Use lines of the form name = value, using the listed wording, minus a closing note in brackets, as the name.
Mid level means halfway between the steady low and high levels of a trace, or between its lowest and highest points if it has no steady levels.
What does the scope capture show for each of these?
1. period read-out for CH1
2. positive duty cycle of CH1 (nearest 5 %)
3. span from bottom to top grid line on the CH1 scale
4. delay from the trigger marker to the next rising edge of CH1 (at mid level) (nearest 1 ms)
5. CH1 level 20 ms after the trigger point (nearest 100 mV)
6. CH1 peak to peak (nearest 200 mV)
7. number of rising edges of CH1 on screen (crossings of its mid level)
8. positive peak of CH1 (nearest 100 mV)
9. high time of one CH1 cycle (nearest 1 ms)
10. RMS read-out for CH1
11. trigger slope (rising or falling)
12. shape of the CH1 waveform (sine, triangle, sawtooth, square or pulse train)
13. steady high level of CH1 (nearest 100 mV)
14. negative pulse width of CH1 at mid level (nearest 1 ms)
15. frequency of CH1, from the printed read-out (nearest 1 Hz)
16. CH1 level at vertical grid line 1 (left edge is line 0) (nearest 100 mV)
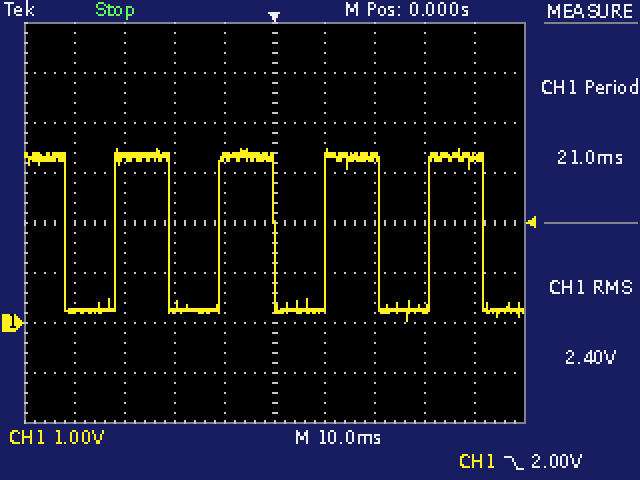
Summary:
period read-out for CH1 = 21.0 ms
positive duty cycle of CH1 = 50 %
span from bottom to top grid line on the CH1 scale = 8 V
delay from the trigger marker to the next rising edge of CH1 (at mid level) = 10 ms
CH1 level 20 ms after the trigger point = 3.3 V
CH1 peak to peak = 3.4 V
number of rising edges of CH1 on screen = 4
positive peak of CH1 = 3.5 V
high time of one CH1 cycle = 11 ms
RMS read-out for CH1 = 2.40 V
trigger slope = falling
shape of the CH1 waveform = square
steady high level of CH1 = 3.3 V
negative pulse width of CH1 at mid level = 10 ms
frequency of CH1, from the printed read-out = 48 Hz
CH1 level at vertical grid line 1 (left edge is line 0) = 200 mV
